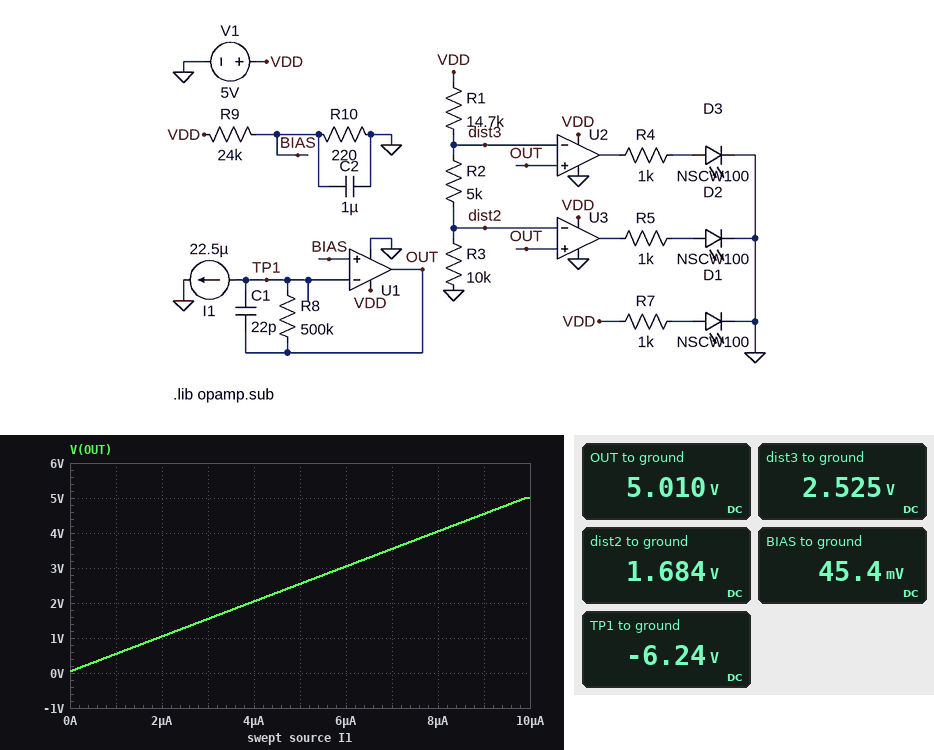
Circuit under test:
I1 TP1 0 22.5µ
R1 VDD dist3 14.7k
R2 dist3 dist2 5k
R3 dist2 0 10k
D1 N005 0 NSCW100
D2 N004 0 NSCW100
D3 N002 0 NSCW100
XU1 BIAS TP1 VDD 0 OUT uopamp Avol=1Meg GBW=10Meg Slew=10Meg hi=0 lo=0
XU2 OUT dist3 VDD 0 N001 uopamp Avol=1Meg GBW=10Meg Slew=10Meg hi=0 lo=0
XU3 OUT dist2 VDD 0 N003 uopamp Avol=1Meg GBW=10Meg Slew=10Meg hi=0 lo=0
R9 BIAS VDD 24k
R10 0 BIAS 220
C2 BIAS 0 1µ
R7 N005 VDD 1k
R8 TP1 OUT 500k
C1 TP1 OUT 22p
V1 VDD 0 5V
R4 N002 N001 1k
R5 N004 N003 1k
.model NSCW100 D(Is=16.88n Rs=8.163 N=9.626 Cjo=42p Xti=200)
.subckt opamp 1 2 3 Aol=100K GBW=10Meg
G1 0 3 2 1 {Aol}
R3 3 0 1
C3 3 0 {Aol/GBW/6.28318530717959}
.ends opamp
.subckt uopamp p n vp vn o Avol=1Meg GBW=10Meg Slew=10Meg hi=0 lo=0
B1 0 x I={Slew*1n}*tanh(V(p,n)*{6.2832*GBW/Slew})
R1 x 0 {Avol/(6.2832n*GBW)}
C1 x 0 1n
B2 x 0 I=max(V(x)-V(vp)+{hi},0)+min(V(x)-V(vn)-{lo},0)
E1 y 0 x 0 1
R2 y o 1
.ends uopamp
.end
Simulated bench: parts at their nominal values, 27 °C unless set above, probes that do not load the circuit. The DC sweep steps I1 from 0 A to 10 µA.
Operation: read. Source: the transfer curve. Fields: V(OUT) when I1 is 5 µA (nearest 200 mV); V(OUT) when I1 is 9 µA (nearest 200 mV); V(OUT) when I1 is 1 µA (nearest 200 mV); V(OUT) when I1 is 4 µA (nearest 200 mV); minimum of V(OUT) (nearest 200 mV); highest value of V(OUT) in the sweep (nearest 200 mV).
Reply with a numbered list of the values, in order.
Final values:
1. 2.6 V
2. 4.6 V
3. 600 mV
4. 2.0 V
5. 0 V
6. 5.0 V
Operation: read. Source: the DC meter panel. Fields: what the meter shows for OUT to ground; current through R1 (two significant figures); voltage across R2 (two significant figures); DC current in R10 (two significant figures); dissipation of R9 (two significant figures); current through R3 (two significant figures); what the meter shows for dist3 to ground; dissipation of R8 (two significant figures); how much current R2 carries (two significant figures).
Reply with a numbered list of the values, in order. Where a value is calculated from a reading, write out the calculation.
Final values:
1. 5.010 V
2. (5 V - 2.525 V) / 14.7 kΩ = 170 µA
3. 2.525 V - 1.684 V = 840 mV
4. (45.4 mV) / 220 Ω = 210 µA
5. (5 V - 45.4 mV)^2 / 24 kΩ = 1.0 mW
6. (1.684 V) / 10 kΩ = 170 µA
7. 2.525 V
8. (5.01 V - (-6.24 V))^2 / 500 kΩ = 250 µW
9. (2.525 V - 1.684 V) / 5 kΩ = 170 µA
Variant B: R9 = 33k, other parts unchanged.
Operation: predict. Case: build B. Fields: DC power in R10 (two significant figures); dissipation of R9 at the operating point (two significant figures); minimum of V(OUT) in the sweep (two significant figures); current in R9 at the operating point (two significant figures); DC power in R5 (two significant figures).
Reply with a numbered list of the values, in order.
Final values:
1. 5.0 µW
2. 750 µW
3. 33 mV
4. 150 µA
5. 4.3 mW
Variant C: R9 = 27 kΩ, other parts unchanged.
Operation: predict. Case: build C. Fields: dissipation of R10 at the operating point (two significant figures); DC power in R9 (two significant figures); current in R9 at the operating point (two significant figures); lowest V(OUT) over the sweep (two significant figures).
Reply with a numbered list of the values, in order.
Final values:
1. 7.4 µW
2. 910 µW
3. 180 µA
4. 40 mV
